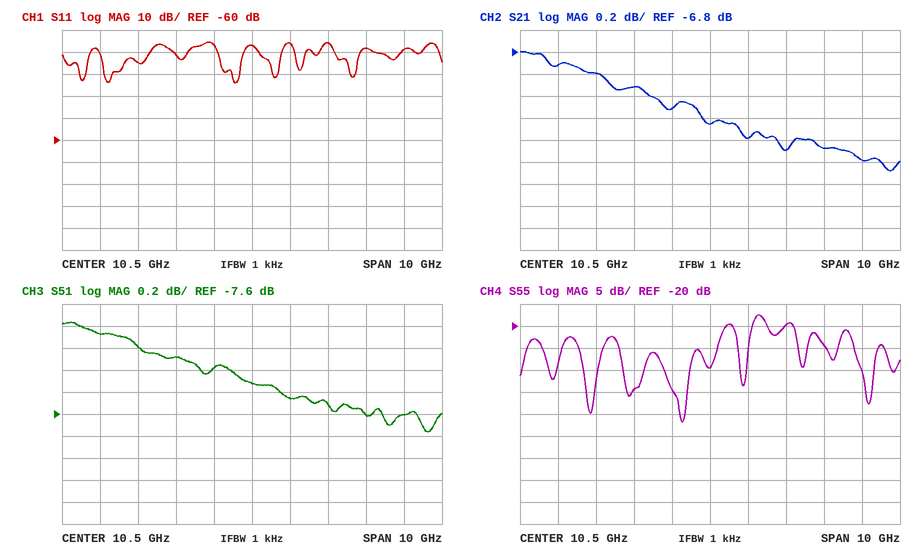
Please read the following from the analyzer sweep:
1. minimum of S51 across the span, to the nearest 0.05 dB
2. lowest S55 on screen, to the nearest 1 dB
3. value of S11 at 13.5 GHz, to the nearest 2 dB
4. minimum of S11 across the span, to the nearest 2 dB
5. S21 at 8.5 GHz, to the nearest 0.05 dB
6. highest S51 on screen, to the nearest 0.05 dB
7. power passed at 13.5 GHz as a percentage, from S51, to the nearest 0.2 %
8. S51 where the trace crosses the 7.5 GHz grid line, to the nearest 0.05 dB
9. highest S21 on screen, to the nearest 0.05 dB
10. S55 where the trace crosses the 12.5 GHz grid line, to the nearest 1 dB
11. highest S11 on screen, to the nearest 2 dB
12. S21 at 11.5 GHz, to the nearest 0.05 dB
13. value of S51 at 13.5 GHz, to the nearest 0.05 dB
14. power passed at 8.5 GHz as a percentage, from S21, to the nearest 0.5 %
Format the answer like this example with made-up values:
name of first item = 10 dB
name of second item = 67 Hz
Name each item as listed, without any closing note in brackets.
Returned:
minimum of S51 across the span, to the nearest 0.05 dB = -7.75 dB
lowest S55 on screen, to the nearest 1 dB = -42 dB
value of S11 at 13.5 GHz, to the nearest 2 dB = -18 dB
minimum of S11 across the span, to the nearest 2 dB = -34 dB
S21 at 8.5 GHz, to the nearest 0.05 dB = -7.10 dB
highest S51 on screen, to the nearest 0.05 dB = -6.75 dB
power passed at 13.5 GHz as a percentage, from S51, to the nearest 0.2 % = 17.4 %
S51 where the trace crosses the 7.5 GHz grid line, to the nearest 0.05 dB = -7.00 dB
highest S21 on screen, to the nearest 0.05 dB = -6.80 dB
S55 where the trace crosses the 12.5 GHz grid line, to the nearest 1 dB = -20 dB
highest S11 on screen, to the nearest 2 dB = -16 dB
S21 at 11.5 GHz, to the nearest 0.05 dB = -7.60 dB
value of S51 at 13.5 GHz, to the nearest 0.05 dB = -7.60 dB
power passed at 8.5 GHz as a percentage, from S21, to the nearest 0.5 % = 19.5 %
